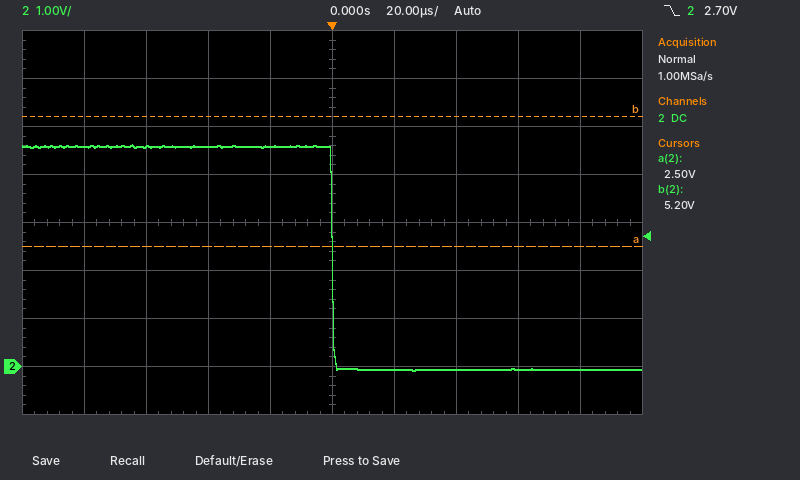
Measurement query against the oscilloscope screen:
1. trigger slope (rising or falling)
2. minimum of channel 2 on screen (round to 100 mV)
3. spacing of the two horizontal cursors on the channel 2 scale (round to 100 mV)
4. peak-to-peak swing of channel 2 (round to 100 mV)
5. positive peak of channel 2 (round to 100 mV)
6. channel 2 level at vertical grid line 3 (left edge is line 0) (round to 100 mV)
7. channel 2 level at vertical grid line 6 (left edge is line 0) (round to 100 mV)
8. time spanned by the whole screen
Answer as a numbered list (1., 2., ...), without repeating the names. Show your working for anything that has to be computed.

1. falling
2. -100 mV
3. 2.7 V
4. 4.6 V − (-100 mV) = 4.7 V
5. 4.6 V
6. 4.6 V
7. -100 mV
8. 200 µs
